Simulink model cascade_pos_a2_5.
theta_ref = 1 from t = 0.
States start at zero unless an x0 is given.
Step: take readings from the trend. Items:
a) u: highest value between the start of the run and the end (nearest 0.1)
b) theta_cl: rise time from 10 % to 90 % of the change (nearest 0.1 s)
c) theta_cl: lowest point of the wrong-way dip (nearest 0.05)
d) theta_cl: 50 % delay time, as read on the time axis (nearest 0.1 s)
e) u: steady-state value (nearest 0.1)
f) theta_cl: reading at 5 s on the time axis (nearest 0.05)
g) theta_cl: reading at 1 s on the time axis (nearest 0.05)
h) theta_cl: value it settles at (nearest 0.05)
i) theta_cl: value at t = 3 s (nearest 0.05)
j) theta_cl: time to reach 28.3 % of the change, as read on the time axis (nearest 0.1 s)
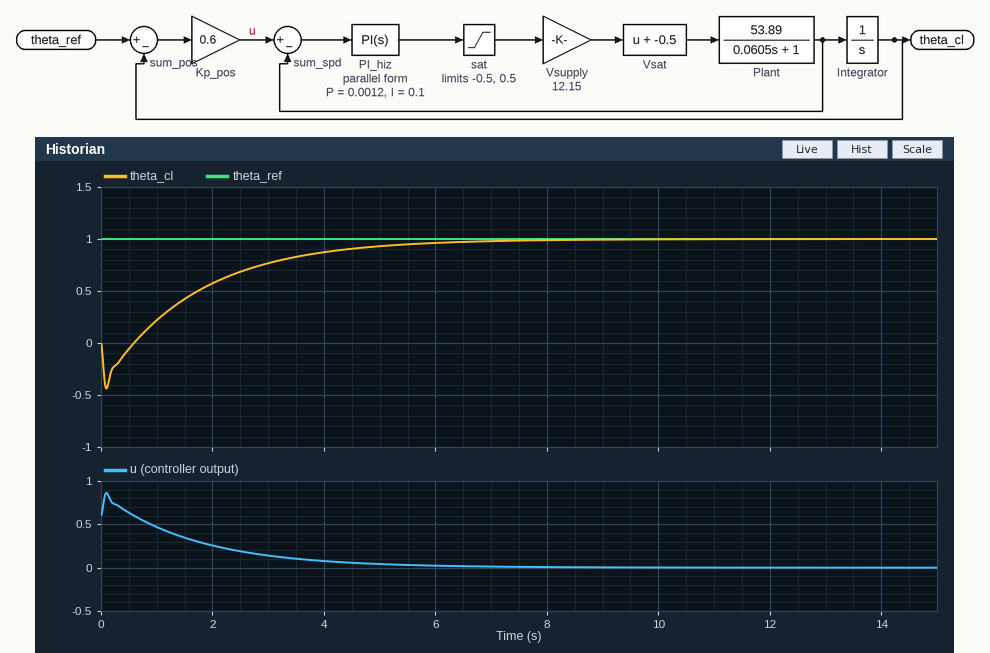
0.9
3.6 s
-0.45
1.7 s
0.0
0.95
0.20
1.00
0.75
1.1 s
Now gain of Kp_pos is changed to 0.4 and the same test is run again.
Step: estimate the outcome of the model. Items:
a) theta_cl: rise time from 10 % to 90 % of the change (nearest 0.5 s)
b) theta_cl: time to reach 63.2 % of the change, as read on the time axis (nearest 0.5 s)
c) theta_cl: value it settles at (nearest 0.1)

5.5 s
3.5 s
1.0
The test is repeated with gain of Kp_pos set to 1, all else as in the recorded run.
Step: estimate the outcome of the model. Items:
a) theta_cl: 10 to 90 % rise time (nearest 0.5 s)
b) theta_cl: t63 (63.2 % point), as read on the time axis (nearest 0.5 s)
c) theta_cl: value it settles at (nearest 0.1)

2.0 s
1.5 s
1.0
